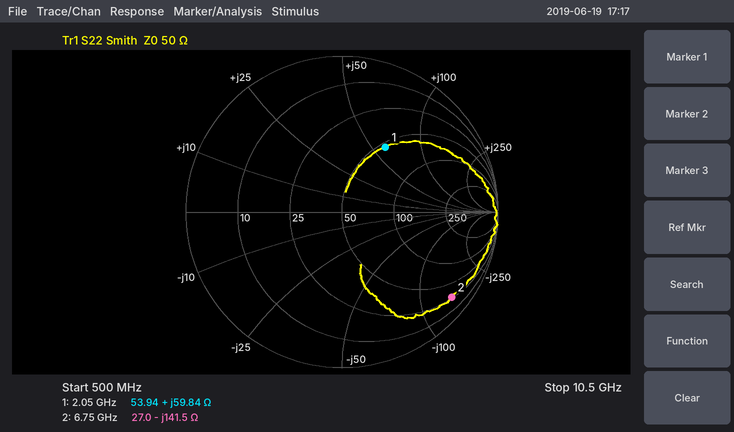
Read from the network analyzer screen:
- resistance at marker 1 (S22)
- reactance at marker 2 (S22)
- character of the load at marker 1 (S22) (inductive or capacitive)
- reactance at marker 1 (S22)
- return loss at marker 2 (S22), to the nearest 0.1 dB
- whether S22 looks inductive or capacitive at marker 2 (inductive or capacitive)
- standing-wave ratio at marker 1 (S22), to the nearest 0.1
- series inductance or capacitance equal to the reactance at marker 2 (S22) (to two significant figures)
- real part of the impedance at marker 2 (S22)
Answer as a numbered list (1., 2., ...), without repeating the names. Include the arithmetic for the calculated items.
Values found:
1. 53.94 Ω
2. -141.5 Ω
3. inductive
4. +59.84 Ω
5. 1.0 dB
6. capacitive
7. 3.0
8. C = 1/(2π × 6.75 GHz × 141.5 Ω) ≈ 167 fF, so 170 fF to two significant figures
9. 27.0 Ω
